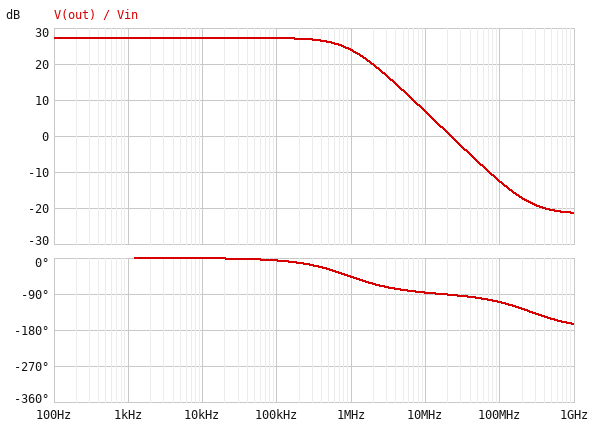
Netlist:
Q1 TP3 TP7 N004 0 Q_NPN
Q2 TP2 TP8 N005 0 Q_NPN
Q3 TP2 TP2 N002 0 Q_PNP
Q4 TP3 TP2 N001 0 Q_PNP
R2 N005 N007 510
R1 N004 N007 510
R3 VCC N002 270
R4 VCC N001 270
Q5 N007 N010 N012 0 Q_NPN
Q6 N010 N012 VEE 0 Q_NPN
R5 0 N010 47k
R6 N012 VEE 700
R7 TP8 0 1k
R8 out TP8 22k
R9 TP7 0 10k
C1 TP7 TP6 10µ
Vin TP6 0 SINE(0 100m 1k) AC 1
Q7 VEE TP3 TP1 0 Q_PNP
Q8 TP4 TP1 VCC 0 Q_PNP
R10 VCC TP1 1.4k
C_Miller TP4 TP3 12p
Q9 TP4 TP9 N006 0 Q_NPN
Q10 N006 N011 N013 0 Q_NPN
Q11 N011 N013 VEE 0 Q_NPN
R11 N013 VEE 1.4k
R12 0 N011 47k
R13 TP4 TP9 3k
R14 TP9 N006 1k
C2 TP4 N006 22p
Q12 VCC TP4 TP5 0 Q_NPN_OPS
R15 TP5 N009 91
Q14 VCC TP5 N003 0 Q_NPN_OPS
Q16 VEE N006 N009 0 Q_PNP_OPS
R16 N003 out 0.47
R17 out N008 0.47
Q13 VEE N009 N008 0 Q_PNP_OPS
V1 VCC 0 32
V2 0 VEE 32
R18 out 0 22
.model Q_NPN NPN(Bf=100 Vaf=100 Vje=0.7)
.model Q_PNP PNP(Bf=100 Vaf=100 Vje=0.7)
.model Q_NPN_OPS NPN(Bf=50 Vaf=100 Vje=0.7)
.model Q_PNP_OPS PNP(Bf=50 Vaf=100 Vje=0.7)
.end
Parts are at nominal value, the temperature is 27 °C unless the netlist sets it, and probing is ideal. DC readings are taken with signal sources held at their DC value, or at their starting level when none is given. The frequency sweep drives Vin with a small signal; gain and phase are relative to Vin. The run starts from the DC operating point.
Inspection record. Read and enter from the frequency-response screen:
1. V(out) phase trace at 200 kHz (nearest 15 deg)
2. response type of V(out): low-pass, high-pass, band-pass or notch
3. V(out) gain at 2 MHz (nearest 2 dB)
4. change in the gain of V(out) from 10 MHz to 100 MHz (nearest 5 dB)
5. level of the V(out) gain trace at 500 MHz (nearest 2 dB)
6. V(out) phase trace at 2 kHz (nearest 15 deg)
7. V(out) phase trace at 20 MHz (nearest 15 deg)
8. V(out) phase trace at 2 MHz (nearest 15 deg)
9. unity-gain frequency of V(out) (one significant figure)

-15 deg
low-pass
20 dB
-20 dB
-20 dB
0 deg
-90 deg
-60 deg
20 MHz
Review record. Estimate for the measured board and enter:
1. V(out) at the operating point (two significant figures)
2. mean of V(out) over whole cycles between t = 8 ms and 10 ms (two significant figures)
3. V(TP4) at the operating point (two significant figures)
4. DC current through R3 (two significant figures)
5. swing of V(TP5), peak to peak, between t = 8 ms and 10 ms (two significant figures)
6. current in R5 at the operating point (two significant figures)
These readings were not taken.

-770 mV
-770 mV
-510 mV
540 µA
6.2 V
650 µA
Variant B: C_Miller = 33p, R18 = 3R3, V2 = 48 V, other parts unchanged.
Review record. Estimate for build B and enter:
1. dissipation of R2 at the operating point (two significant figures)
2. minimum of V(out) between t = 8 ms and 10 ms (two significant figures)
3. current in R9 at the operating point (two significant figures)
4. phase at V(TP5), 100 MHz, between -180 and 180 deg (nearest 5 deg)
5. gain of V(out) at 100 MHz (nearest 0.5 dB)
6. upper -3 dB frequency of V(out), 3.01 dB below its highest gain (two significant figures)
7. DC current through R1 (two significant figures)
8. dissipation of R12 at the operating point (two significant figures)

160 µW
-3.1 V
4.2 µA
-135 deg
-19.5 dB
270 kHz
550 µA
46 mW
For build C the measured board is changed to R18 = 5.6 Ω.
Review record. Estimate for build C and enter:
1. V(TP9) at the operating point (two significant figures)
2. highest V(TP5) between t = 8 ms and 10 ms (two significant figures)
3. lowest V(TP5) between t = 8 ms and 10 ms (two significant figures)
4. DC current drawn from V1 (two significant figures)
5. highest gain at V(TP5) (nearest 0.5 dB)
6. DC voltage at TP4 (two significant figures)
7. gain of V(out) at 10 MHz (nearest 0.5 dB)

-2.1 V
2.6 V
-4.2 V
5.1 mA
29.0 dB
-660 mV
6.0 dB
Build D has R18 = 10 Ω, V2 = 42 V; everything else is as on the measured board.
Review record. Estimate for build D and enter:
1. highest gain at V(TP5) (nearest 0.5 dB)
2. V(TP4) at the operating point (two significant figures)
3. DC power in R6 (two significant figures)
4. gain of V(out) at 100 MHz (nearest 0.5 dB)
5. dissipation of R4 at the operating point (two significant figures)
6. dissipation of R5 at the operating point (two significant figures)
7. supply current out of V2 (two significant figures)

28.5 dB
-550 mV
850 µW
-13.0 dB
80 µW
35 mW
85 mA
